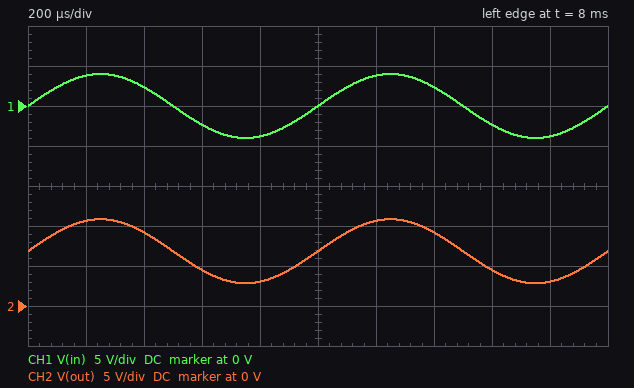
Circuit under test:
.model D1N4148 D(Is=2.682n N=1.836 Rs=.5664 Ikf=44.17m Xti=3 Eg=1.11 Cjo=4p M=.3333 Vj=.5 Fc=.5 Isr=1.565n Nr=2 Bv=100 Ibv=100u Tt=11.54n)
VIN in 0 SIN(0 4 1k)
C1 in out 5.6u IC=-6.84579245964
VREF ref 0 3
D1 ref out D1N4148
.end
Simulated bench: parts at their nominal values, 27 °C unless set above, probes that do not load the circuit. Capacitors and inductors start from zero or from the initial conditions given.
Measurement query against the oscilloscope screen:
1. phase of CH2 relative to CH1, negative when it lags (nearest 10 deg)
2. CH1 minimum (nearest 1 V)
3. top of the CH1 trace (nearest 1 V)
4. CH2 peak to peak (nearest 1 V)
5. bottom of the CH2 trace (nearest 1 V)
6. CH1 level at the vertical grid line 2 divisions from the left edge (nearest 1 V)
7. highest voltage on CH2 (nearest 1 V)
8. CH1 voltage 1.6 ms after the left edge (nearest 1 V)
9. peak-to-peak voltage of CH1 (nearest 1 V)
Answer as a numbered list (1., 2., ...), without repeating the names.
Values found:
1. 0 deg
2. -4 V
3. 4 V
4. 8 V
5. 3 V
6. 2 V
7. 11 V
8. -2 V
9. 8 V
